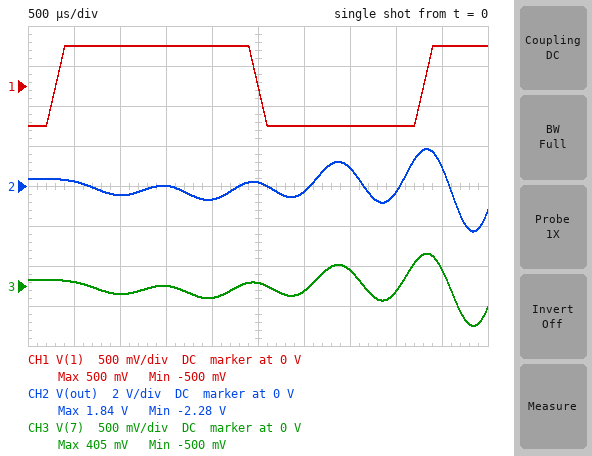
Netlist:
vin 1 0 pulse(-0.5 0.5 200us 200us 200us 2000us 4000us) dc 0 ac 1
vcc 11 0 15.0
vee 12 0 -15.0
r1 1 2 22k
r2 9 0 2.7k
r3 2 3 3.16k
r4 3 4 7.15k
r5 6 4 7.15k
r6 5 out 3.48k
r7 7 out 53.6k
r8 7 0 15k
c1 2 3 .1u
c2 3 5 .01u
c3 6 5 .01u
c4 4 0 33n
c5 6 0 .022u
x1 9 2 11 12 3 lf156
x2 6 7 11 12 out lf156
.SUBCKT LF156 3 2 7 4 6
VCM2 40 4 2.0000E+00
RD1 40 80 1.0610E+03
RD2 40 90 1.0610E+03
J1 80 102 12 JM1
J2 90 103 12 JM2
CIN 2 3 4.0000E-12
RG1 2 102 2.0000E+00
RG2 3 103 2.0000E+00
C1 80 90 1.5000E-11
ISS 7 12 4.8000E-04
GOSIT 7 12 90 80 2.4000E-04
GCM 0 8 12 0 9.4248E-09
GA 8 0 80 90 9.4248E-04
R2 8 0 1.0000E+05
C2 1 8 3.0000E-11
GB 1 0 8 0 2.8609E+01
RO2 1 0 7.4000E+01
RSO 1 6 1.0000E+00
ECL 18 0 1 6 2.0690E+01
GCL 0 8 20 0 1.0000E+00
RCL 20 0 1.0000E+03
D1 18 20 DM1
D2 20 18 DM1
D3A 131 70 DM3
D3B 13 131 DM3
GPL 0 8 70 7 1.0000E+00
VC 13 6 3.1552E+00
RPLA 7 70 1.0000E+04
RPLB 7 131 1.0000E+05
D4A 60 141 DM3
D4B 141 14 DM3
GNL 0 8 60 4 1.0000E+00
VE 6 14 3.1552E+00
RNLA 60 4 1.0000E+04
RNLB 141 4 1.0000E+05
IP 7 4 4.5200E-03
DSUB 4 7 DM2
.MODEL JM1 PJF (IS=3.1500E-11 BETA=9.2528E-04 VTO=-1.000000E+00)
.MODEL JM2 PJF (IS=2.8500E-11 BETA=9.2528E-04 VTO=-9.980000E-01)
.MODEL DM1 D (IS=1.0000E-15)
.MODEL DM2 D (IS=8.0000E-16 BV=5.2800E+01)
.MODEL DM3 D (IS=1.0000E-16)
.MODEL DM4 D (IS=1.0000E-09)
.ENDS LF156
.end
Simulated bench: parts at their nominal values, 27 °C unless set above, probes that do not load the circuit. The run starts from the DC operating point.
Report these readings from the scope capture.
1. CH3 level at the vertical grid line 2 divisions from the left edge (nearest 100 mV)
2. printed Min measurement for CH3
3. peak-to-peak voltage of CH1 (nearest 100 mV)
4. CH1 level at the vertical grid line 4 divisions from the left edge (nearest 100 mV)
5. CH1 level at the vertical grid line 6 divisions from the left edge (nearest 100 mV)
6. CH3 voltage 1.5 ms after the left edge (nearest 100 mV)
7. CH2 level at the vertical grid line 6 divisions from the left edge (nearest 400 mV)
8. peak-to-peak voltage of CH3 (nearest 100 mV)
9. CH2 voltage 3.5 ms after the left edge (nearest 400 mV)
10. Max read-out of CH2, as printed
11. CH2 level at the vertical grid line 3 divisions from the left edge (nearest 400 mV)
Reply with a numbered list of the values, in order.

1. -100 mV
2. -500 mV
3. 1.0 V
4. 500 mV
5. -500 mV
6. 0 V
7. -400 mV
8. 900 mV
9. 800 mV
10. 1.84 V
11. 0 V
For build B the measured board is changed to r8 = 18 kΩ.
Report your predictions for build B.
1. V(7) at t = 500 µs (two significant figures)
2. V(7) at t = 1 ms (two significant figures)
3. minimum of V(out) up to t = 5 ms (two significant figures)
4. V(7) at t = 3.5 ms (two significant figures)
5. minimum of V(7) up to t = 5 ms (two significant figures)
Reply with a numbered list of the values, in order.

1. 55 mV
2. -61 mV
3. -290 mV
4. 71 mV
5. -72 mV
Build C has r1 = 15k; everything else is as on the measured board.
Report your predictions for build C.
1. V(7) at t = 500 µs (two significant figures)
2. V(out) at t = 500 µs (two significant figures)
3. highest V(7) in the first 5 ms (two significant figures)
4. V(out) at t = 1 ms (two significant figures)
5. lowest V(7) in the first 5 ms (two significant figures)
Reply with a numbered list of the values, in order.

1. 71 mV
2. 320 mV
3. 590 mV
4. -690 mV
5. -730 mV
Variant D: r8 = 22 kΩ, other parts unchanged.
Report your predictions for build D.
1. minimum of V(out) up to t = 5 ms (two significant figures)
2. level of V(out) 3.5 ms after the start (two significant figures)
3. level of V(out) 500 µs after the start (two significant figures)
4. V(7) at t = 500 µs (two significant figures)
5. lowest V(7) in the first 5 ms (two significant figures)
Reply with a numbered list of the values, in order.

1. -230 mV
2. 230 mV
3. 200 mV
4. 59 mV
5. -67 mV
